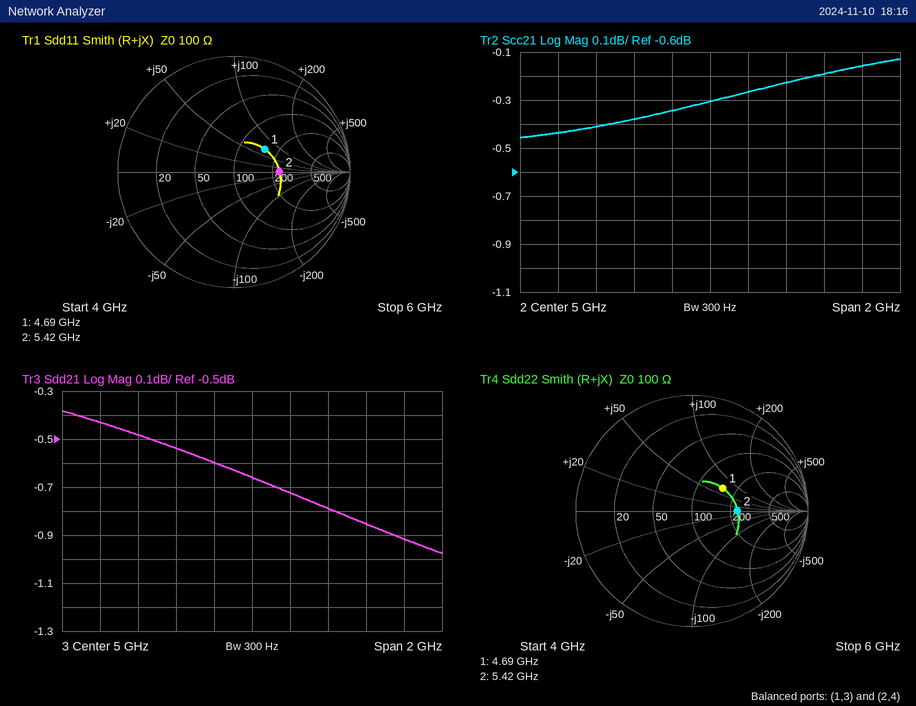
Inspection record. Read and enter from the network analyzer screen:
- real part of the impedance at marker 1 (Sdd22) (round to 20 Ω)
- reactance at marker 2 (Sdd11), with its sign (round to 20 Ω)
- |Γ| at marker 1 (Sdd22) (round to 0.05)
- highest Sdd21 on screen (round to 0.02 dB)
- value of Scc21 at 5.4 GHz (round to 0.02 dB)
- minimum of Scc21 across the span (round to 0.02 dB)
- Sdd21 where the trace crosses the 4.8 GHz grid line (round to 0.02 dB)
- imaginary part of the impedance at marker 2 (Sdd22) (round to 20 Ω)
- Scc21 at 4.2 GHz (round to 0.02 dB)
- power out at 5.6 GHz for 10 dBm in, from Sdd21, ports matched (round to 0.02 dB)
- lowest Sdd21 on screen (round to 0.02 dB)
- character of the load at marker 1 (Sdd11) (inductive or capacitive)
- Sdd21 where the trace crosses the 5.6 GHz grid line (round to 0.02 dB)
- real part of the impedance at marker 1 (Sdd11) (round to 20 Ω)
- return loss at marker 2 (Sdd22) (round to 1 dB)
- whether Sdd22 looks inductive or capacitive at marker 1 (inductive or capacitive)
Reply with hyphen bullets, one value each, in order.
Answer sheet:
- 160 Ω
- 0 Ω
- 0.35
- -0.38 dB
- -0.22 dB
- -0.46 dB
- -0.60 dB
- 0 Ω
- -0.44 dB
- 9.14 dBm
- -0.98 dB
- inductive
- -0.86 dB
- 160 Ω
- 8 dB
- inductive
